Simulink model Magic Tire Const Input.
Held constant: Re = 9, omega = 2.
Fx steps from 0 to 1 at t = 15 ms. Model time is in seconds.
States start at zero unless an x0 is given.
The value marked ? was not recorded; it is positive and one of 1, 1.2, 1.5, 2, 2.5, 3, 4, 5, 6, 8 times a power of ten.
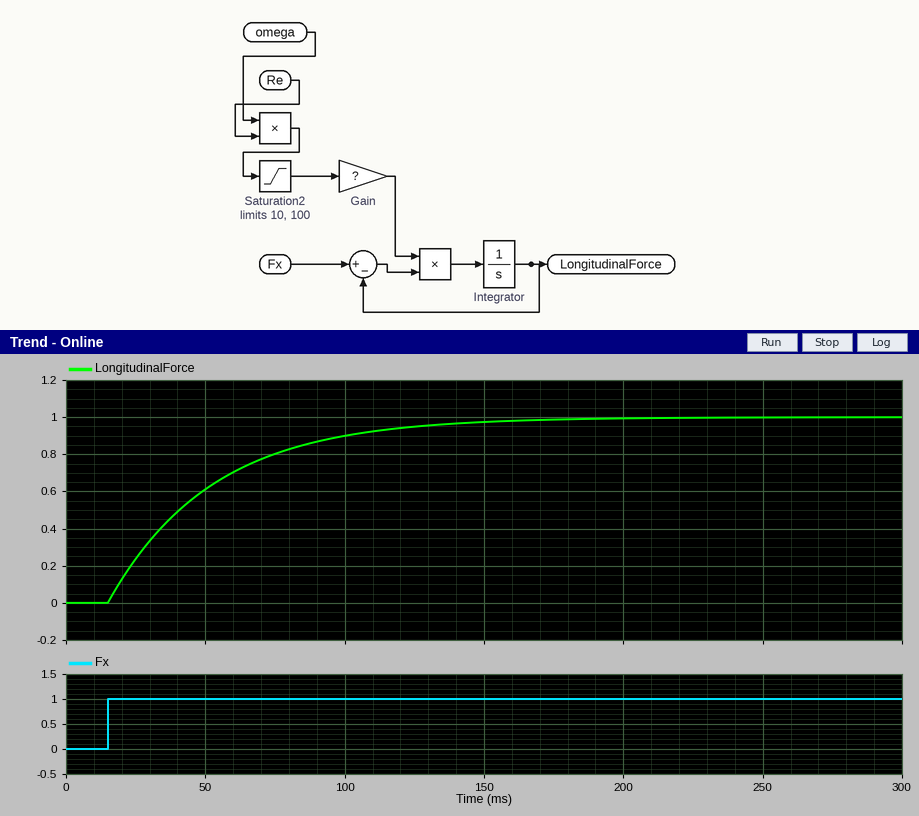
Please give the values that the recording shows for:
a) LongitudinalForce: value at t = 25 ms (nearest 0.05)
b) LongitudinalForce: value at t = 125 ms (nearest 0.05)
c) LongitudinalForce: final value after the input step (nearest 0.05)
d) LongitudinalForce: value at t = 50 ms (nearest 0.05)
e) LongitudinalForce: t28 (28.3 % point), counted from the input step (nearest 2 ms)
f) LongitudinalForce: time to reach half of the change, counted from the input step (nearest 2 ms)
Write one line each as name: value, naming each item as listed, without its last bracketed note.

LongitudinalForce: value at t = 25 ms: 0.25
LongitudinalForce: value at t = 125 ms: 0.95
LongitudinalForce: final value after the input step: 1.00
LongitudinalForce: value at t = 50 ms: 0.60
LongitudinalForce: t28 (28.3 % point), counted from the input step: 12 ms
LongitudinalForce: time to reach half of the change, counted from the input step: 26 ms
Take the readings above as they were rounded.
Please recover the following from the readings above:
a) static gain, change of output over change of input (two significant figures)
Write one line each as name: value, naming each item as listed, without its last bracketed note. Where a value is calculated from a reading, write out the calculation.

static gain, change of output over change of input: (1 - 0) / (1 - 0) = 1.0
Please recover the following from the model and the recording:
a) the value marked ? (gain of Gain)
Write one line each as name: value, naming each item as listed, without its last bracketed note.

the value marked ?: 1.5
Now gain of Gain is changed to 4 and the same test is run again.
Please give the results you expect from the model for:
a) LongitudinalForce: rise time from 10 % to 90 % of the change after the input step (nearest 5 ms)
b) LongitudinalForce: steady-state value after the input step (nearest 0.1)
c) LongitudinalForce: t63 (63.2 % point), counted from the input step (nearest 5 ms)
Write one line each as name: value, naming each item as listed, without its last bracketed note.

LongitudinalForce: rise time from 10 % to 90 % of the change after the input step: 30 ms
LongitudinalForce: steady-state value after the input step: 1.0
LongitudinalForce: t63 (63.2 % point), counted from the input step: 15 ms
